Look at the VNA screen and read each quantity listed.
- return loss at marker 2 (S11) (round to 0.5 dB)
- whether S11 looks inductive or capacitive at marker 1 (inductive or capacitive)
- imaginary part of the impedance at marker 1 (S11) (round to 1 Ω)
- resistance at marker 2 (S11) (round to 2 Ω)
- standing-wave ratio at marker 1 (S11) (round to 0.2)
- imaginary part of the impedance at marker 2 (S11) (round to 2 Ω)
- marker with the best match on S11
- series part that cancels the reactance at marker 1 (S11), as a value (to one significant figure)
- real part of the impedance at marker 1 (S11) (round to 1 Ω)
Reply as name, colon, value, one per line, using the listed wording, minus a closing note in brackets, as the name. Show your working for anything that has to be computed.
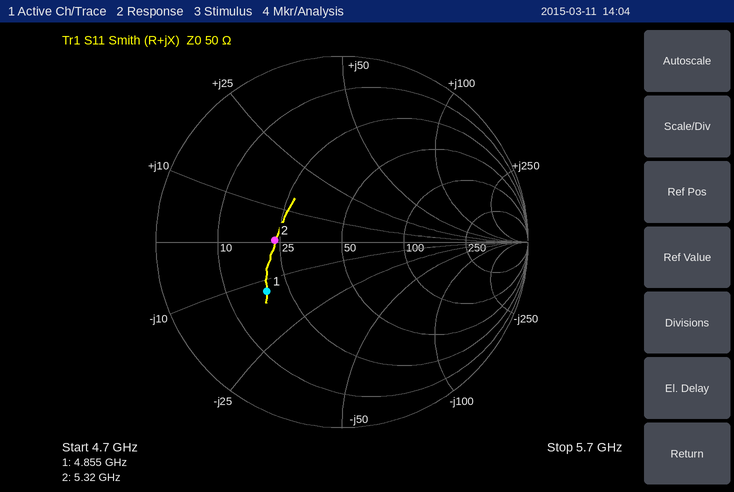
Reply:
return loss at marker 2 (S11): 9.0 dB
whether S11 looks inductive or capacitive at marker 1: capacitive
imaginary part of the impedance at marker 1 (S11): -13 Ω
resistance at marker 2 (S11): 24 Ω
standing-wave ratio at marker 1 (S11): 2.8
imaginary part of the impedance at marker 2 (S11): 0 Ω
marker with the best match on S11: marker 2
series part that cancels the reactance at marker 1 (S11), as a value: L = 13 Ω/(2π × 4.855 GHz) ≈ 426 pH, so 400 pH to one significant figure
real part of the impedance at marker 1 (S11): 19 Ω
